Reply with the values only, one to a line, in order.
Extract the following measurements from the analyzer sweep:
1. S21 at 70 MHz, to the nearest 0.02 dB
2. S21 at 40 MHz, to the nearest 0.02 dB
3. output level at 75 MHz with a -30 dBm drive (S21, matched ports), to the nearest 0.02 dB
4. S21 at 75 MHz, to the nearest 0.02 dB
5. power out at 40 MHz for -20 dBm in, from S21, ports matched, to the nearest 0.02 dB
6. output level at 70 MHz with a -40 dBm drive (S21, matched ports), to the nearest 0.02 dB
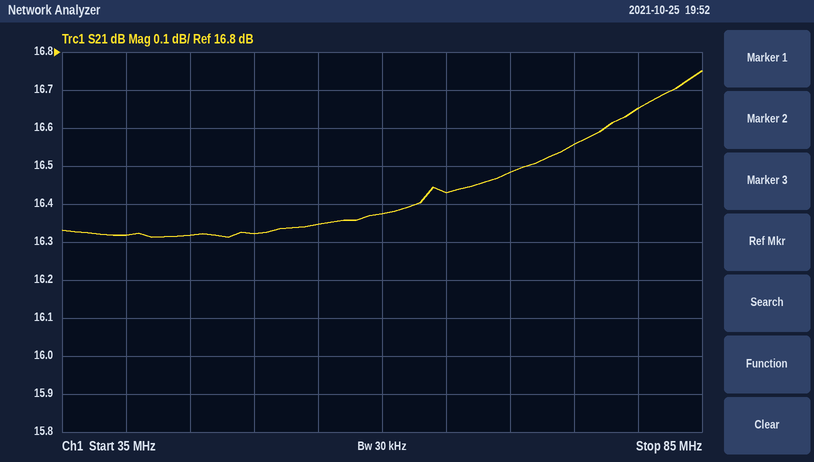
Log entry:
16.48 dB
16.32 dB
-13.44 dBm
16.56 dB
-3.68 dBm
-23.52 dBm
